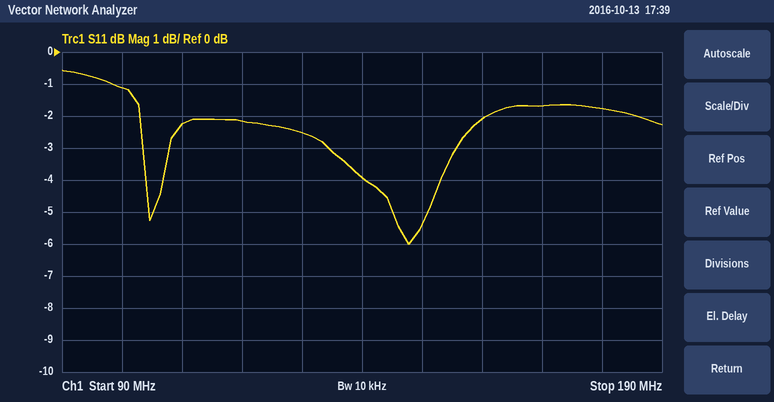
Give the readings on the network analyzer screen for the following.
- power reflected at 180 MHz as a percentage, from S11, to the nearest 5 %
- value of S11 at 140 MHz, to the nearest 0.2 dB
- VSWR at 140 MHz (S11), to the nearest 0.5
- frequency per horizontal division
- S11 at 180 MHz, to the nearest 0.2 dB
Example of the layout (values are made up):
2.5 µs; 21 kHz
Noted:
65 %; -4.0 dB; 4.5; 10 MHz; -1.8 dB
